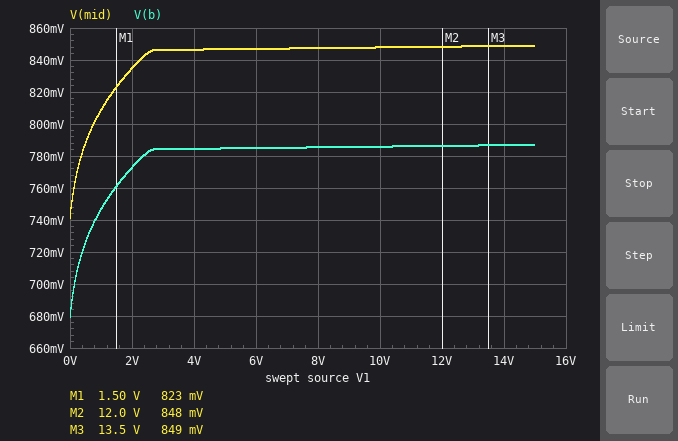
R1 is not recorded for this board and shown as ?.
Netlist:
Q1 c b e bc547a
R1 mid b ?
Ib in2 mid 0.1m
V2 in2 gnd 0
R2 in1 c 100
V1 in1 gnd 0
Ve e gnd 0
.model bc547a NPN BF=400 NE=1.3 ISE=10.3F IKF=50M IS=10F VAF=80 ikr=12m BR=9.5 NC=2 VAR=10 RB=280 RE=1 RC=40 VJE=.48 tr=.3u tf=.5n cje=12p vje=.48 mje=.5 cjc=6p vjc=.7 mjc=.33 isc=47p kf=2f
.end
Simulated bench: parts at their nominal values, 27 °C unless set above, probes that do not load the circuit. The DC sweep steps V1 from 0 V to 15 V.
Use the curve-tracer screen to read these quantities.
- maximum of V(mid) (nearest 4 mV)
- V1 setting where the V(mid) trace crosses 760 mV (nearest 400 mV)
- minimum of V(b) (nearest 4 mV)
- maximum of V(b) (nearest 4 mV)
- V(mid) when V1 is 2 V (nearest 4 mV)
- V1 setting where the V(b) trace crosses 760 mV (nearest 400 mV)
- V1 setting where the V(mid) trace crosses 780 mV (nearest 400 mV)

848 mV
0 V
680 mV
788 mV
836 mV
1.6 V
400 mV
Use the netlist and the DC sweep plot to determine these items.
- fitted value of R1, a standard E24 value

620 Ω
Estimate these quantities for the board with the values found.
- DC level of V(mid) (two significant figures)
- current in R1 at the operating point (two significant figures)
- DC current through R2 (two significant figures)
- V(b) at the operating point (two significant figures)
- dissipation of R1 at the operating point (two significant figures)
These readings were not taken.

740 mV
100 µA
20 µA
680 mV
6.2 µW
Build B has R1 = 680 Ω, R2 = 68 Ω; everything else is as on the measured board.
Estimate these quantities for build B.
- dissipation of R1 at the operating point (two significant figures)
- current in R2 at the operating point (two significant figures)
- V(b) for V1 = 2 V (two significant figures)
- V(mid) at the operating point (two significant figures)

6.8 µW
25 µA
780 mV
750 mV
